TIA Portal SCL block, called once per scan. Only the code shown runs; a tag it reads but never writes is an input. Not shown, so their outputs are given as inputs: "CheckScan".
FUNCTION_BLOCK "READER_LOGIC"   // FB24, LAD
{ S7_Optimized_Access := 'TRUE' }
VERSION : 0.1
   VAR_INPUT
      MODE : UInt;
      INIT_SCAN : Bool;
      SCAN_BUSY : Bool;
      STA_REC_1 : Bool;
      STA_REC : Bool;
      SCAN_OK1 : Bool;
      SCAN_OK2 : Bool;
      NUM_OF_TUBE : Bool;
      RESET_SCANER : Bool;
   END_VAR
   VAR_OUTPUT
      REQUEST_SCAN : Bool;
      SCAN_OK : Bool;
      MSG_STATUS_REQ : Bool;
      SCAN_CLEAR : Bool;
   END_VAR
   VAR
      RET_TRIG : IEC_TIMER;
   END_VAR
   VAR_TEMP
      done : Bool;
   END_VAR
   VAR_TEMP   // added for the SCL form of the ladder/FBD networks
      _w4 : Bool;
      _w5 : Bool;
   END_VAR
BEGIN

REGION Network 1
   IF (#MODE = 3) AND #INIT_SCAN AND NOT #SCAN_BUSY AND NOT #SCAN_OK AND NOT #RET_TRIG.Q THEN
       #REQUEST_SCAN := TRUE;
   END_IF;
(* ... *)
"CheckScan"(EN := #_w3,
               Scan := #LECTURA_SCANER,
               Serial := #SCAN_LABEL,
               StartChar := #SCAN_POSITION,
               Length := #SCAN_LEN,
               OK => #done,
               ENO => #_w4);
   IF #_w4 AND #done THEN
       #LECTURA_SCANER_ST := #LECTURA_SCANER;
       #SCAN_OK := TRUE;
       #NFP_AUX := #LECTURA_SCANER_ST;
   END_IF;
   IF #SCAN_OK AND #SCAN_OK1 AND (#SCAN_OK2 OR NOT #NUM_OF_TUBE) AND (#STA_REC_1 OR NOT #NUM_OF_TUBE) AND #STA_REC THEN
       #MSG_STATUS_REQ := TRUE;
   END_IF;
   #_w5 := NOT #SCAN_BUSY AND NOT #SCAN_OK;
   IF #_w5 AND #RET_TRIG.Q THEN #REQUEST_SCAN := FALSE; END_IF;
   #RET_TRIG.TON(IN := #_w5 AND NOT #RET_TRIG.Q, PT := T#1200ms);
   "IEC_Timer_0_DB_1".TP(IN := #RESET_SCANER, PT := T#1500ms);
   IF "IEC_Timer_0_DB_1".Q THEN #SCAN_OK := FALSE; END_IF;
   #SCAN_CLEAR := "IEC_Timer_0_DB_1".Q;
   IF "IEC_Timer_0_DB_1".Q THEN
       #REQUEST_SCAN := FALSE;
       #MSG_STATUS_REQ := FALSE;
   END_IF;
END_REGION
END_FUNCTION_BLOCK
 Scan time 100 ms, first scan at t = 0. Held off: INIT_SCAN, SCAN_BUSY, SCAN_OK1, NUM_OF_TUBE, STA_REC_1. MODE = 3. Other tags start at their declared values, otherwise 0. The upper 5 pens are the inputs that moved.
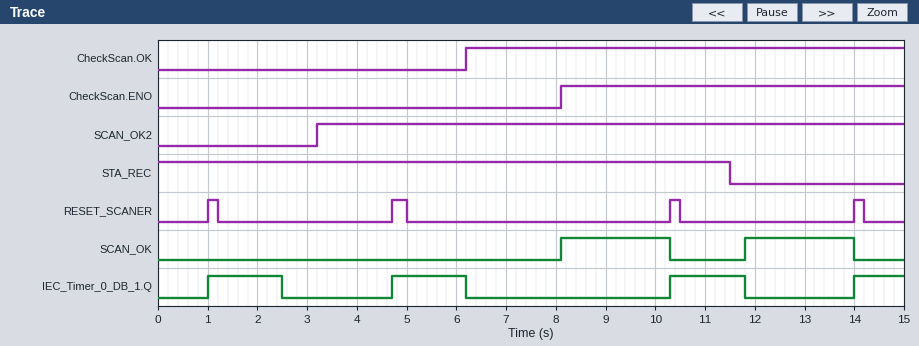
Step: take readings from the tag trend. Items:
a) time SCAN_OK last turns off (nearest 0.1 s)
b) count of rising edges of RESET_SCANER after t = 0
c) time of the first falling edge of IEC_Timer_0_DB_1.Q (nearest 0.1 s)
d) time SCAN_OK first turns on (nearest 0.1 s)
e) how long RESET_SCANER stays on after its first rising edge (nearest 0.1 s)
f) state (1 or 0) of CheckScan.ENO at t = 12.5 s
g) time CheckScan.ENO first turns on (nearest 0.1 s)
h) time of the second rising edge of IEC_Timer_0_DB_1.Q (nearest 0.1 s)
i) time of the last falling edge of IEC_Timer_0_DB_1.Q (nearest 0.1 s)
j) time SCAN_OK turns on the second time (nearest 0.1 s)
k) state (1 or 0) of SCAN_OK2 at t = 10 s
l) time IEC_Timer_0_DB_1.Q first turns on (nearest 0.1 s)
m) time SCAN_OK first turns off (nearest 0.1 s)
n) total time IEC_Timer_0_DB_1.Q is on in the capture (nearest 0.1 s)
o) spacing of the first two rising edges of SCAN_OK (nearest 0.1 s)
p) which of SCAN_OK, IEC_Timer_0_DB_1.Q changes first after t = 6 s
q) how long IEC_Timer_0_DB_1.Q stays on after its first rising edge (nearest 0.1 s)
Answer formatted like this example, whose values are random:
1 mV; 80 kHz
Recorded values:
14.0 s; 4; 2.5 s; 8.1 s; 0.2 s; 1; 8.1 s; 4.7 s; 11.8 s; 11.8 s; 1; 1.0 s; 10.3 s; 5.5 s; 3.7 s; IEC_Timer_0_DB_1.Q; 1.5 s
